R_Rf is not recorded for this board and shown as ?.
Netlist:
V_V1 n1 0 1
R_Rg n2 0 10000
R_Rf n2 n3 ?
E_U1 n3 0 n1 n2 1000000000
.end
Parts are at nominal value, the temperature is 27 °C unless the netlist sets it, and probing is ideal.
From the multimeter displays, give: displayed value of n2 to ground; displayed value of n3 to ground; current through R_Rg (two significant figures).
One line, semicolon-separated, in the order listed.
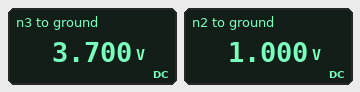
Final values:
1.000 V; 3.700 V; 100 µA
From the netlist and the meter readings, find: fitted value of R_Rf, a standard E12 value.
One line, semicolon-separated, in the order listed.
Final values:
27 kΩ
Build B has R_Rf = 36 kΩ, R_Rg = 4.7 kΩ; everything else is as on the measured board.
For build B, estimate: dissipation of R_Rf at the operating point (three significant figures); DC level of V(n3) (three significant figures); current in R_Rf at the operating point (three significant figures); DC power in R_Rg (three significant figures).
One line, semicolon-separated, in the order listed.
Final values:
1.63 mW; 8.66 V; 213 µA; 213 µW
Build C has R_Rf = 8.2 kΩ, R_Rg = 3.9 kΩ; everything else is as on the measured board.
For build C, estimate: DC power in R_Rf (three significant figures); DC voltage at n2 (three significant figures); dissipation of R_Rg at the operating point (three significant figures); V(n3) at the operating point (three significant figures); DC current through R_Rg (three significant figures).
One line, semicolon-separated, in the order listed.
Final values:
539 µW; 1.00 V; 256 µW; 3.10 V; 256 µA
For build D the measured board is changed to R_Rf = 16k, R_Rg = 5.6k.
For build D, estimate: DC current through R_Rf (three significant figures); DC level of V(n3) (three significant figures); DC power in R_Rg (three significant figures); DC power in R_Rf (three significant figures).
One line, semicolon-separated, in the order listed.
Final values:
179 µA; 3.86 V; 179 µW; 510 µW
